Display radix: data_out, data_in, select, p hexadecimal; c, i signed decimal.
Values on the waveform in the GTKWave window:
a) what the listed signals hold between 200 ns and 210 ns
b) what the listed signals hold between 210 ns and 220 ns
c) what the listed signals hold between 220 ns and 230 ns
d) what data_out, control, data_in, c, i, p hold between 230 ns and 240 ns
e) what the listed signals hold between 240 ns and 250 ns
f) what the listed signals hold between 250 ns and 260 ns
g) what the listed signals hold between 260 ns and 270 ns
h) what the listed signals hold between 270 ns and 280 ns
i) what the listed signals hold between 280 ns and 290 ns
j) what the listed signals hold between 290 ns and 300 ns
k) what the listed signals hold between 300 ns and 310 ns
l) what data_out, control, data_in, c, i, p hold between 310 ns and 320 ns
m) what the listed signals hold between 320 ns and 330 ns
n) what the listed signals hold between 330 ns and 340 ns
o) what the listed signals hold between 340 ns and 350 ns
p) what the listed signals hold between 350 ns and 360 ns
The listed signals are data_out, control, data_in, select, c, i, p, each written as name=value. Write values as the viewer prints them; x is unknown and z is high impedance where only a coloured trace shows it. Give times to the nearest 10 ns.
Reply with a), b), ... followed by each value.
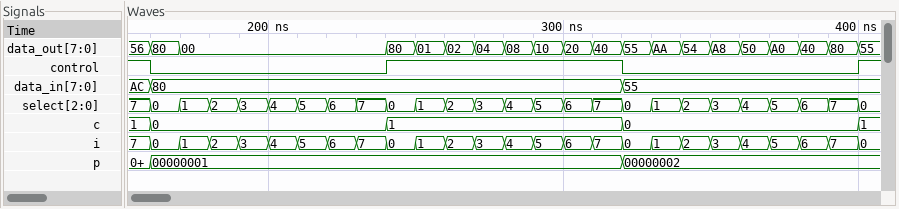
a) data_out=00, control=0, data_in=80, select=4, c=0, i=4, p=00000001
b) data_out=00, control=0, data_in=80, select=5, c=0, i=5, p=00000001
c) data_out=00, control=0, data_in=80, select=6, c=0, i=6, p=00000001
d) data_out=00, control=0, data_in=80, c=0, i=7, p=00000001
e) data_out=80, control=1, data_in=80, select=0, c=1, i=0, p=00000001
f) data_out=01, control=1, data_in=80, select=1, c=1, i=1, p=00000001
g) data_out=02, control=1, data_in=80, select=2, c=1, i=2, p=00000001
h) data_out=04, control=1, data_in=80, select=3, c=1, i=3, p=00000001
i) data_out=08, control=1, data_in=80, select=4, c=1, i=4, p=00000001
j) data_out=10, control=1, data_in=80, select=5, c=1, i=5, p=00000001
k) data_out=20, control=1, data_in=80, select=6, c=1, i=6, p=00000001
l) data_out=40, control=1, data_in=80, c=1, i=7, p=00000001
m) data_out=55, control=0, data_in=55, select=0, c=0, i=0, p=00000002
n) data_out=AA, control=0, data_in=55, select=1, c=0, i=1, p=00000002
o) data_out=54, control=0, data_in=55, select=2, c=0, i=2, p=00000002
p) data_out=A8, control=0, data_in=55, select=3, c=0, i=3, p=00000002
